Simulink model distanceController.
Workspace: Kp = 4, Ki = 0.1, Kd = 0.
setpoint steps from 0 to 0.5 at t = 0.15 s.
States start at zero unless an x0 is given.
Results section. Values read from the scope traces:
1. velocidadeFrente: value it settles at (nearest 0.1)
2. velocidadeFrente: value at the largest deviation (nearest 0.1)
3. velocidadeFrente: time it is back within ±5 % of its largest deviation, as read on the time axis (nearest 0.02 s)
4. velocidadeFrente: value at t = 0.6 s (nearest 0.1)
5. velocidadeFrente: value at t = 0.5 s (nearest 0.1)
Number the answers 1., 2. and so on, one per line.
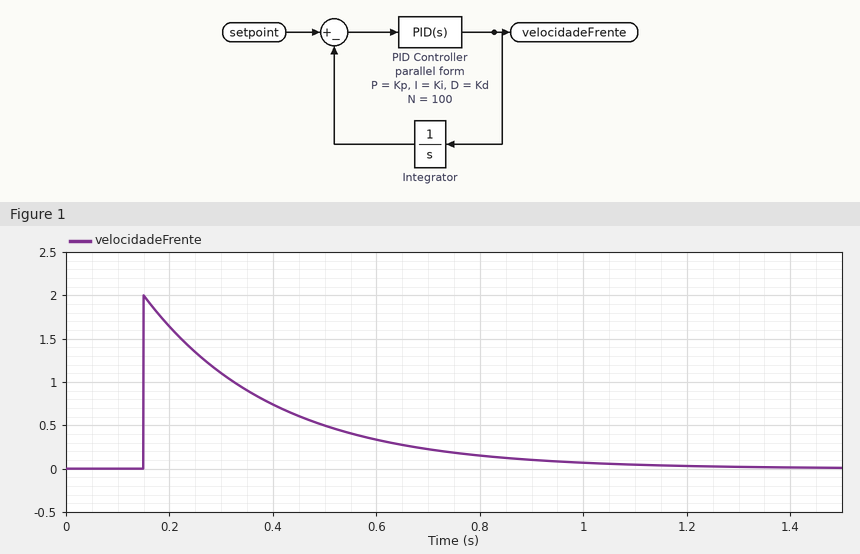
1. 0.0
2. 2.0
3. 0.90 s
4. 0.3
5. 0.5
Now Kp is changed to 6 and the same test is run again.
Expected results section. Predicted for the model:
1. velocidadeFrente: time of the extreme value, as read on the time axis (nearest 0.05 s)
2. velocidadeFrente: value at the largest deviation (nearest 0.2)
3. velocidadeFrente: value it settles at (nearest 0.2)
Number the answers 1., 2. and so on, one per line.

1. 0.15 s
2. 3.0
3. 0.0
